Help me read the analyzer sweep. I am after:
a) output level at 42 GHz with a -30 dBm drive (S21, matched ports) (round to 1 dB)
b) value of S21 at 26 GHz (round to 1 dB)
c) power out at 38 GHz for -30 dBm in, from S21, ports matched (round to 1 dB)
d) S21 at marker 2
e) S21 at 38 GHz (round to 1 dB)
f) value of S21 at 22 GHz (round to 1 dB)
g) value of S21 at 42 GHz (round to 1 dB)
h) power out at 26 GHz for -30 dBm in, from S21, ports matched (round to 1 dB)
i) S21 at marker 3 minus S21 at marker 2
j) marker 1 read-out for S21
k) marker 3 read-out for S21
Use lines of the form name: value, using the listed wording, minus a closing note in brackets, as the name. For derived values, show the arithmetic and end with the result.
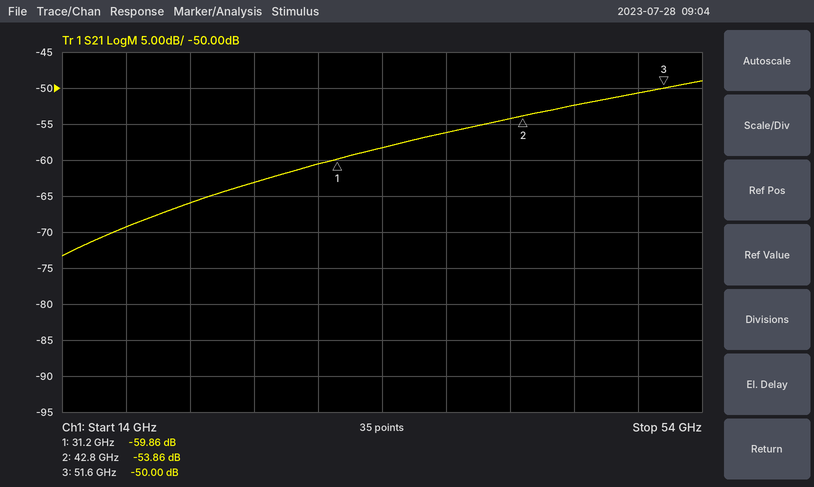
output level at 42 GHz with a -30 dBm drive (S21, matched ports): -30 dBm + (-54 dB) = -84 dBm
value of S21 at 26 GHz: -63 dB
power out at 38 GHz for -30 dBm in, from S21, ports matched: -30 dBm + (-56 dB) = -86 dBm
S21 at marker 2: -53.86 dB
S21 at 38 GHz: -56 dB
value of S21 at 22 GHz: -66 dB
value of S21 at 42 GHz: -54 dB
power out at 26 GHz for -30 dBm in, from S21, ports matched: -30 dBm + (-63 dB) = -93 dBm
S21 at marker 3 minus S21 at marker 2: -50 − (-53.86) = 3.86 dB
marker 1 read-out for S21: -59.86 dB
marker 3 read-out for S21: -50.00 dB
